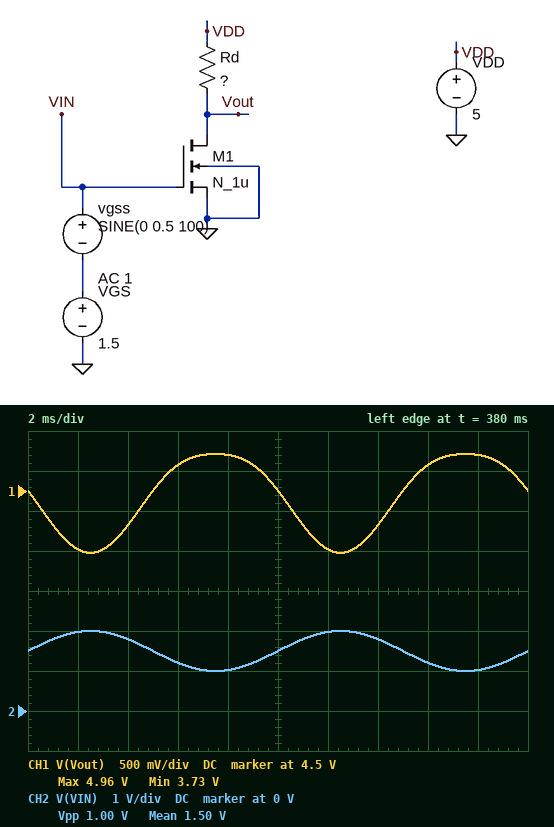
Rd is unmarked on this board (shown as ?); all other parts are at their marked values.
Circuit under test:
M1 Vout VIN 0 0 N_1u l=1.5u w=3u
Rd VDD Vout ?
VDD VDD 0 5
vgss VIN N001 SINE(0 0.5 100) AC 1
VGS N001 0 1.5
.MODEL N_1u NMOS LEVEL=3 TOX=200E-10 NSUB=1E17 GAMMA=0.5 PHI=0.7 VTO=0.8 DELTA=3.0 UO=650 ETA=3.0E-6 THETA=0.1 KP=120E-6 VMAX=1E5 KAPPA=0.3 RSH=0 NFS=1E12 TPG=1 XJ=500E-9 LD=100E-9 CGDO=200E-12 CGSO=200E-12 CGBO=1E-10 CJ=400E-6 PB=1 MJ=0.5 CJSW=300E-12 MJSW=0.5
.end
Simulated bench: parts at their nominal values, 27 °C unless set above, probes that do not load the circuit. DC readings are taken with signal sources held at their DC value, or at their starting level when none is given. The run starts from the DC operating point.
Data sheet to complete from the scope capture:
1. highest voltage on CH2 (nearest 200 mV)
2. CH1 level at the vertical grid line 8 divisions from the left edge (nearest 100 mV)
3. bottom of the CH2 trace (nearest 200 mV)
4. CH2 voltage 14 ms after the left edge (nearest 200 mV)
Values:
2.0 V
4.8 V
1.0 V
1.8 V
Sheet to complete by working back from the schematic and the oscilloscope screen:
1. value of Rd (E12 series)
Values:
12 kΩ
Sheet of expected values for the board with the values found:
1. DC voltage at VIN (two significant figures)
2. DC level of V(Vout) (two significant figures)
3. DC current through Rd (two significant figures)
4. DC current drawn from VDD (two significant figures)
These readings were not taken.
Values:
1.5 V
4.5 V
41 µA
41 µA
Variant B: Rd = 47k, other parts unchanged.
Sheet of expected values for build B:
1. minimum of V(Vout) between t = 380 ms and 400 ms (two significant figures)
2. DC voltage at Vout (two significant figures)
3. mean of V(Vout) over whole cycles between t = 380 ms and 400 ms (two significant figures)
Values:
600 mV
3.1 V
2.9 V
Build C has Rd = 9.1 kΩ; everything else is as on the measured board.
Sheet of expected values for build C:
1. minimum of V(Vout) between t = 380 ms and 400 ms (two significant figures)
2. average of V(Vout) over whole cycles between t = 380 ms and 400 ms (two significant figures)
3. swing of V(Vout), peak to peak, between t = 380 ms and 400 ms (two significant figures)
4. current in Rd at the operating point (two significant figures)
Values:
4.0 V
4.6 V
940 mV
41 µA
